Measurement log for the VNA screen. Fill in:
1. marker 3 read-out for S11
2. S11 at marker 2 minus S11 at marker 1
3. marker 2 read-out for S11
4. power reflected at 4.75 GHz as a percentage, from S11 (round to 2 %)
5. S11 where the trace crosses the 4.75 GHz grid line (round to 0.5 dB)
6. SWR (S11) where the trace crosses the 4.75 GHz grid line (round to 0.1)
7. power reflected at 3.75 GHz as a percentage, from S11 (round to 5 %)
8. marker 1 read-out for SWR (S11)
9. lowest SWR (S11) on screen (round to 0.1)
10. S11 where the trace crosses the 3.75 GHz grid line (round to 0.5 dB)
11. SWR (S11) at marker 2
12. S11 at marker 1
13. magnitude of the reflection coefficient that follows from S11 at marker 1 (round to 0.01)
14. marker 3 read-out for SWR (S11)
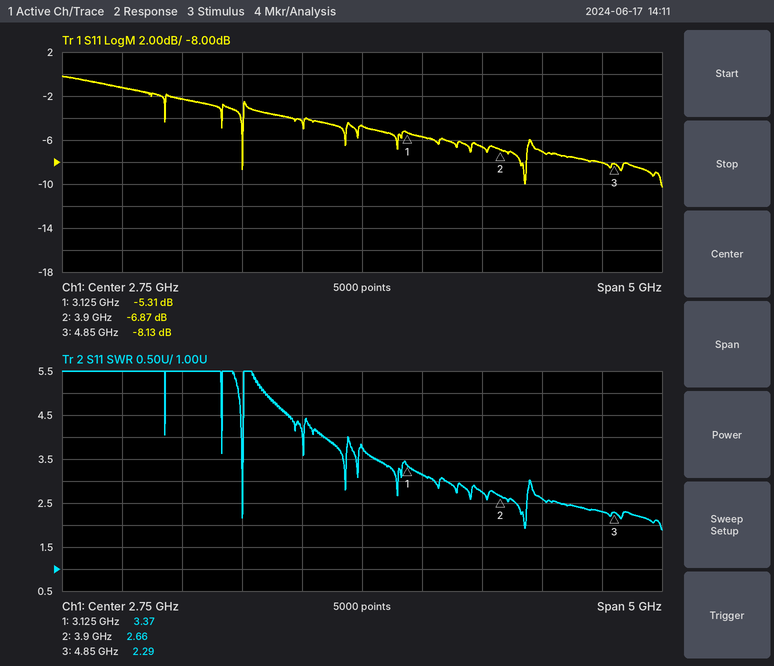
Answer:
-8.13 dB
-1.56 dB
-6.87 dB
16 %
-8.0 dB
2.3
20 %
3.37
1.9
-6.5 dB
2.66
-5.31 dB
0.54
2.29
